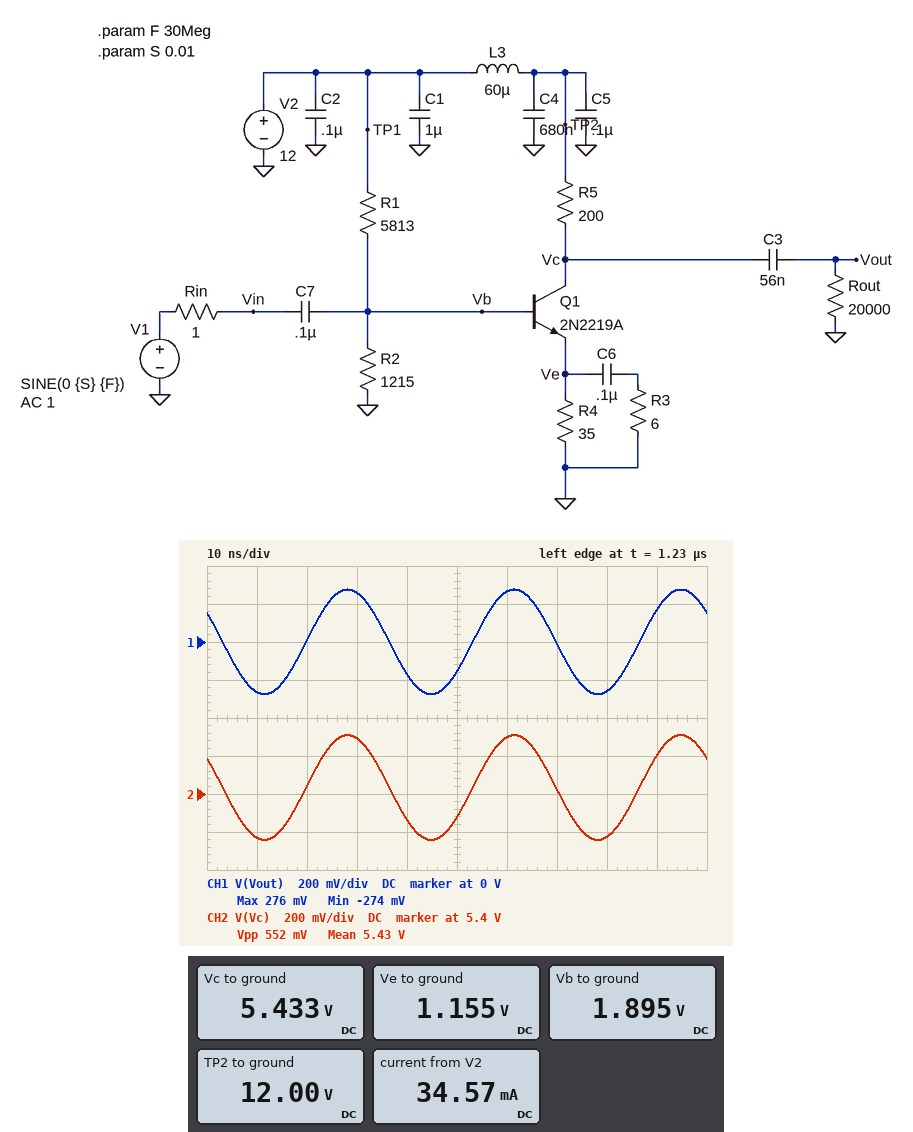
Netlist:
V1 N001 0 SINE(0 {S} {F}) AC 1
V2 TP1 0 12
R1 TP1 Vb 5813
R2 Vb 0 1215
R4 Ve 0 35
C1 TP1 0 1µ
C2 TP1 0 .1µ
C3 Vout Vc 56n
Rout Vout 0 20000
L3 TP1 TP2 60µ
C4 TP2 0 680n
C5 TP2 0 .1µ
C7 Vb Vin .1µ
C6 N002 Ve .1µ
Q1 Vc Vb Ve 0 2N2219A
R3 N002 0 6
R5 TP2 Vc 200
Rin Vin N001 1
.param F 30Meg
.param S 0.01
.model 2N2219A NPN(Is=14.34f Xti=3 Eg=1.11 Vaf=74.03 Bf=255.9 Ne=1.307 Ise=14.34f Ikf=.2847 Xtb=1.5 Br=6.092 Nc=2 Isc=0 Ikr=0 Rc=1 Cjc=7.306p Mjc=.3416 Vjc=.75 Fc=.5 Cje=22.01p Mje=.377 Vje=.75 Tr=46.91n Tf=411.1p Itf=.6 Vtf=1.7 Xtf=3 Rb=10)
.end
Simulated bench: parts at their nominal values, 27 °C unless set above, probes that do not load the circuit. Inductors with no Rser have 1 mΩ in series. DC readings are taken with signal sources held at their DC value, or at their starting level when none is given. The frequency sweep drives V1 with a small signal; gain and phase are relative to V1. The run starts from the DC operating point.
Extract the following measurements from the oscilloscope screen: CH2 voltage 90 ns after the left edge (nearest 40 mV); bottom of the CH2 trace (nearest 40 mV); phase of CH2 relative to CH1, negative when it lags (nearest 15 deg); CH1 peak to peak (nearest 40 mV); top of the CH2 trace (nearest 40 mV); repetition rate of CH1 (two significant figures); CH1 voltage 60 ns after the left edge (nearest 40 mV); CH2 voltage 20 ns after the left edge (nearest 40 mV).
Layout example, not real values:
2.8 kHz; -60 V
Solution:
5.60 V; 5.16 V; 0 deg; 560 mV; 5.72 V; 30 MHz; 280 mV; 5.44 V
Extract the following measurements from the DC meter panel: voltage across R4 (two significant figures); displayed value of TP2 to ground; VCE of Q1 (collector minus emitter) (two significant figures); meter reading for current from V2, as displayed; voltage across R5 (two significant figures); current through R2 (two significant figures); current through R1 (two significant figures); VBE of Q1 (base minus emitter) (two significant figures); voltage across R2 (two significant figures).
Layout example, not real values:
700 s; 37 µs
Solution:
1.2 V; 12.00 V; 4.3 V; 34.57 mA; 6.6 V; 1.6 mA; 1.7 mA; 740 mV; 1.9 V
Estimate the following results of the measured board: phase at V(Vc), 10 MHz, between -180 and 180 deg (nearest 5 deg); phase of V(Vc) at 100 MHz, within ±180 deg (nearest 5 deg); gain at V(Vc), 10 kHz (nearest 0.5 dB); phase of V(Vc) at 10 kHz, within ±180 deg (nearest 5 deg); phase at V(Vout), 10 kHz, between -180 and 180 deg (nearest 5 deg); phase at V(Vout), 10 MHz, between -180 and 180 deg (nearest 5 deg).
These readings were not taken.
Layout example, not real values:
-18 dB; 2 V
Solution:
170 deg; 105 deg; 15.0 dB; -155 deg; -155 deg; 170 deg
